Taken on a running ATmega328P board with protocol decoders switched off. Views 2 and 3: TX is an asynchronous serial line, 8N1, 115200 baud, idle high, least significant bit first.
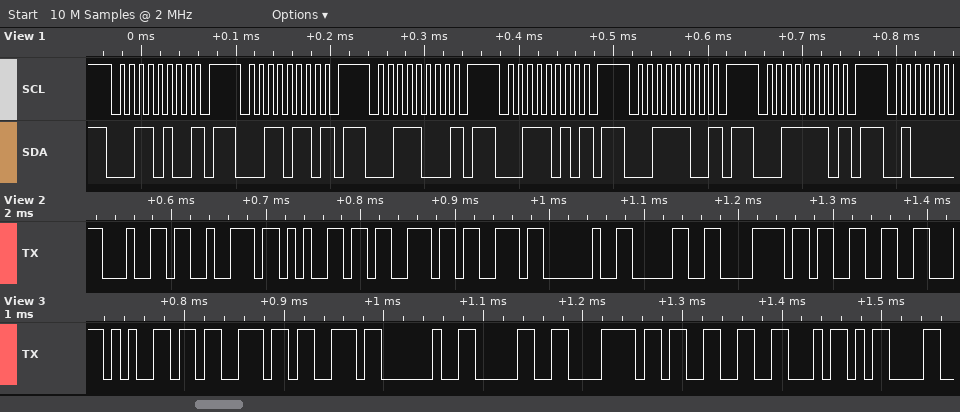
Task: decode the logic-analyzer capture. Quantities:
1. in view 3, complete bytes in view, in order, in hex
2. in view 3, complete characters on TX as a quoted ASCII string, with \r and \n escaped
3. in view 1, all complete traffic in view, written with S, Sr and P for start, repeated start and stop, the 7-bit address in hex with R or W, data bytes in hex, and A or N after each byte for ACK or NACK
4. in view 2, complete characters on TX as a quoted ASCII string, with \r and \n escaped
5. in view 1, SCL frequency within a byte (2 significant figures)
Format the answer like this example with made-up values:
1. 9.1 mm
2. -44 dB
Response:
1. 65 73 73 20 30 78 33 46 0D
2. "ess 0x3F\r"
3. S 1AW N P S 1BW N P S 1CW N P S 1DW N P S 1EW N P S 1FW N P
4. "dress 0x3"
5. 100 kHz
